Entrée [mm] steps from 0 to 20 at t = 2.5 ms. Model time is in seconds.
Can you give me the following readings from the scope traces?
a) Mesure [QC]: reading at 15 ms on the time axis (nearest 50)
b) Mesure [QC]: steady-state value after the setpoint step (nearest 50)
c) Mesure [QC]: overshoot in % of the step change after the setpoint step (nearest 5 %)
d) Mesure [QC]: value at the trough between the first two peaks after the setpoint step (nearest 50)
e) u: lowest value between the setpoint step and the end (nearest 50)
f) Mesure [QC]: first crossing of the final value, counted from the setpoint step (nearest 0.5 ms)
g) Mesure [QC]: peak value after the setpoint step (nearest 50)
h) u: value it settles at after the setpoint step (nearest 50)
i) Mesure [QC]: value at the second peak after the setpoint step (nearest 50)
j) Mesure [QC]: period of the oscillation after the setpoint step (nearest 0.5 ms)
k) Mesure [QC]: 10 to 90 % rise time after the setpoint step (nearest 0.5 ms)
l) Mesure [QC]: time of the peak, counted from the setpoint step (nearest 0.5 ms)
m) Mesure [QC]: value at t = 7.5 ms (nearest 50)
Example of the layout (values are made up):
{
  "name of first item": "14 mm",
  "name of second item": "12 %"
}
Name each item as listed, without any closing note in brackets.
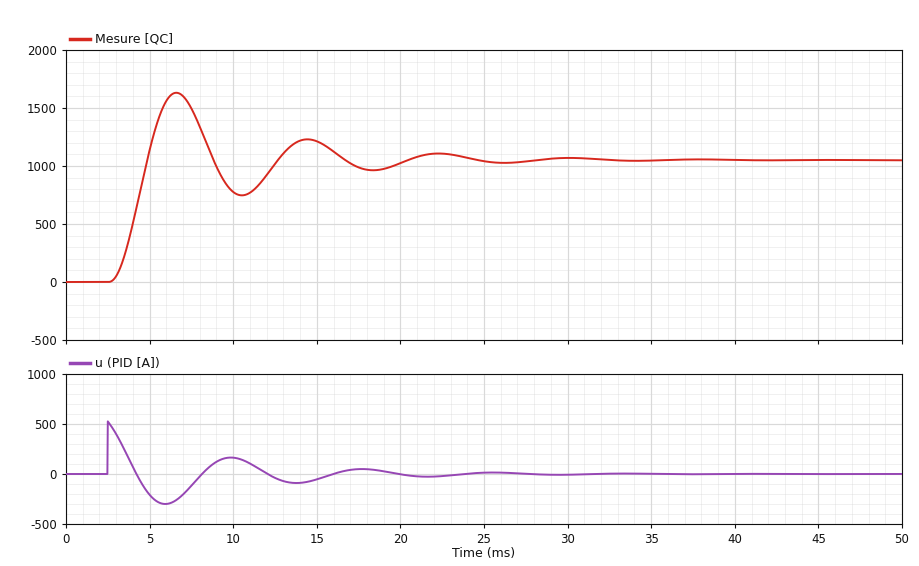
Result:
{
  "Mesure [QC]: reading at 15 ms on the time axis": "1200",
  "Mesure [QC]: steady-state value after the setpoint step": "1050",
  "Mesure [QC]: overshoot in % of the step change after the setpoint step": "55 %",
  "Mesure [QC]: value at the trough between the first two peaks after the setpoint step": "750",
  "u: lowest value between the setpoint step and the end": "-300",
  "Mesure [QC]: first crossing of the final value, counted from the setpoint step": "2.5 ms",
  "Mesure [QC]: peak value after the setpoint step": "1650",
  "u: value it settles at after the setpoint step": "0",
  "Mesure [QC]: value at the second peak after the setpoint step": "1250",
  "Mesure [QC]: period of the oscillation after the setpoint step": "8.0 ms",
  "Mesure [QC]: 10 to 90 % rise time after the setpoint step": "1.5 ms",
  "Mesure [QC]: time of the peak, counted from the setpoint step": "4.0 ms",
  "Mesure [QC]: value at t = 7.5 ms": "1500"
}
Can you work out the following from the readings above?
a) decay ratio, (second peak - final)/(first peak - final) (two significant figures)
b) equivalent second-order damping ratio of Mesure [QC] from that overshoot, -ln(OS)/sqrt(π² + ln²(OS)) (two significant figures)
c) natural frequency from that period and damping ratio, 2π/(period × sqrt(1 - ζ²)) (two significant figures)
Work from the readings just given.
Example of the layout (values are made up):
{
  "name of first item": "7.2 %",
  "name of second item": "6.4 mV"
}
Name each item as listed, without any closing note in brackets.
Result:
{
  "decay ratio, (second peak - final)/(first peak - final)": "0.33",
  "equivalent second-order damping ratio of Mesure [QC] from that overshoot, -ln(OS)/sqrt(π² + ln²(OS))": "0.19",
  "natural frequency from that period and damping ratio, 2π/(period × sqrt(1 - ζ²))": "0.80 rad/ms"
}
